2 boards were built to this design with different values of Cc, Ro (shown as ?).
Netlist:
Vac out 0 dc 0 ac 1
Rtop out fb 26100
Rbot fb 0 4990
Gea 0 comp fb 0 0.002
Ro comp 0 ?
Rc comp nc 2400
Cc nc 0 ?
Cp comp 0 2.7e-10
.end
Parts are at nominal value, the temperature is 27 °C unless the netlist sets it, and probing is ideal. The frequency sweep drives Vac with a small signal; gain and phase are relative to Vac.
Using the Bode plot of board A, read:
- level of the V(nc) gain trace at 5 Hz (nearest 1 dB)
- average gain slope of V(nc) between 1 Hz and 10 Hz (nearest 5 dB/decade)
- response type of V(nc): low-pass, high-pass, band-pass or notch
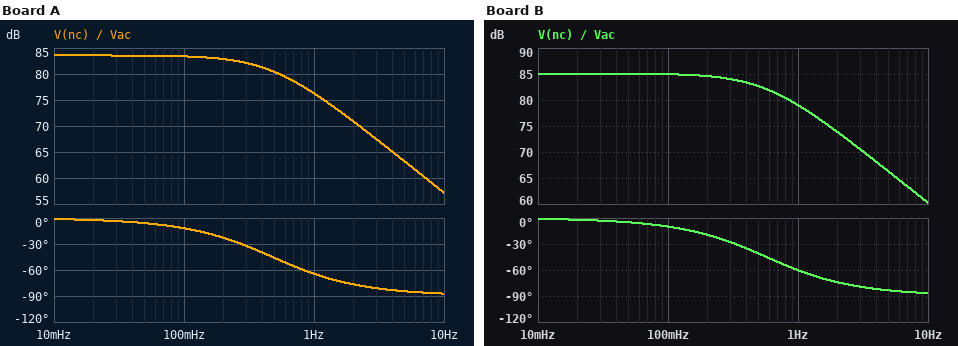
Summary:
63 dB
-20 dB/decade
low-pass
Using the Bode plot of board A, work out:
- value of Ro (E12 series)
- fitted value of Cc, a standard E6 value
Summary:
47 MΩ
6.8 nF
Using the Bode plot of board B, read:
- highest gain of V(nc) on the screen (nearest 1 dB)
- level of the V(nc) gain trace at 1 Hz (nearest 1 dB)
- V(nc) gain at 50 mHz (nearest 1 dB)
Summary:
85 dB
79 dB
85 dB
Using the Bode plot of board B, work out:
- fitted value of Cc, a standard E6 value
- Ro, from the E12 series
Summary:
4.7 nF
56 MΩ
